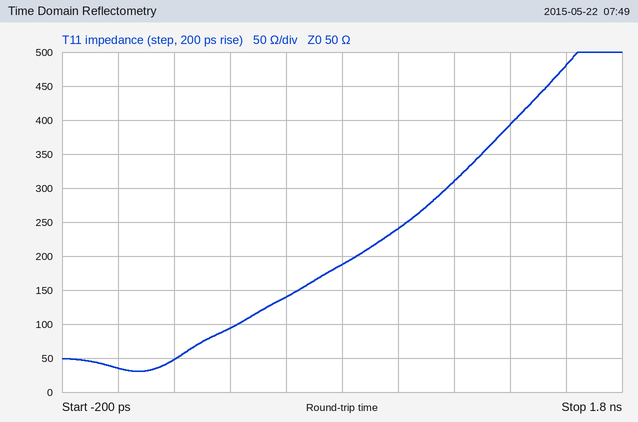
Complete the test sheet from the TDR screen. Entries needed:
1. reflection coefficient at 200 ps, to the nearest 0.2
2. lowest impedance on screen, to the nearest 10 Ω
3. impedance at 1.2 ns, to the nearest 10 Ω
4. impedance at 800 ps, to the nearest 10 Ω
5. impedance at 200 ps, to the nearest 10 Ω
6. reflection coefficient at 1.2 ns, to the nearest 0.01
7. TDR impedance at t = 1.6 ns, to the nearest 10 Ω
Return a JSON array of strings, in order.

["0.0", "30 Ω", "310 Ω", "190 Ω", "50 Ω", "+0.72", "480 Ω"]
